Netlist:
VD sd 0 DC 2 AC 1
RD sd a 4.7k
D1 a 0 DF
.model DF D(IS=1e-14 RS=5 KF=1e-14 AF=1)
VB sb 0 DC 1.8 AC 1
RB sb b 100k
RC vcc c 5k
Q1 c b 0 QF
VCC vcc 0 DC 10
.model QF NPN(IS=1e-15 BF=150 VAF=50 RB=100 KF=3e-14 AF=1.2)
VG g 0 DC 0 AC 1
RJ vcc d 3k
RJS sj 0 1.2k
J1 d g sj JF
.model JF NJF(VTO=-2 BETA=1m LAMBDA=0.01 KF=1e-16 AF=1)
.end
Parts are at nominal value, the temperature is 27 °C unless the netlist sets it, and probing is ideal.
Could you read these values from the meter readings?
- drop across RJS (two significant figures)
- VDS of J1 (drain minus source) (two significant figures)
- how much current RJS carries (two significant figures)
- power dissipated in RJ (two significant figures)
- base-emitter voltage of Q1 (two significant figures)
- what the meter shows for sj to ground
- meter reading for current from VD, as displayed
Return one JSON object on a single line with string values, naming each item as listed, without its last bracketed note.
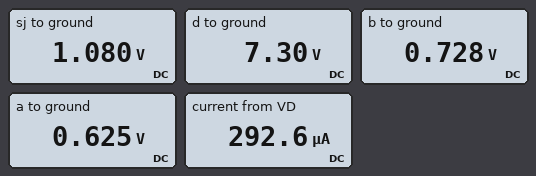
{"drop across RJS": "1.1 V", "VDS of J1 (drain minus source)": "6.2 V", "how much current RJS carries": "900 µA", "power dissipated in RJ": "2.4 mW", "base-emitter voltage of Q1": "730 mV", "what the meter shows for sj to ground": "1.080 V", "meter reading for current from VD, as displayed": "292.6 µA"}
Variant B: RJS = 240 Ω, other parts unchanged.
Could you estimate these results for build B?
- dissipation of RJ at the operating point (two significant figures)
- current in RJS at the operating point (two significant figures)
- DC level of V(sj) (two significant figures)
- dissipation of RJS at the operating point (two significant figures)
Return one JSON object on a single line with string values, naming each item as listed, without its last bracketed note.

{"dissipation of RJ at the operating point": "15 mW", "current in RJS at the operating point": "2.2 mA", "DC level of V(sj)": "530 mV", "dissipation of RJS at the operating point": "1.2 mW"}
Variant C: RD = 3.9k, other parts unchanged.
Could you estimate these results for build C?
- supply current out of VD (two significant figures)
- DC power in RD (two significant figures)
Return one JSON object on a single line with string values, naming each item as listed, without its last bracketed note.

{"supply current out of VD": "350 µA", "DC power in RD": "480 µW"}
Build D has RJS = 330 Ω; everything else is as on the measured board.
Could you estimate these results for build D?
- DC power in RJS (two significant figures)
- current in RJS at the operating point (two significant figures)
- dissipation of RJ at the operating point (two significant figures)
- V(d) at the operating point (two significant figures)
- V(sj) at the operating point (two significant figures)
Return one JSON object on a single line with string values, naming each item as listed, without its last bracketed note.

{"DC power in RJS": "1.2 mW", "current in RJS at the operating point": "1.9 mA", "dissipation of RJ at the operating point": "11 mW", "V(d) at the operating point": "4.2 V", "V(sj) at the operating point": "640 mV"}
